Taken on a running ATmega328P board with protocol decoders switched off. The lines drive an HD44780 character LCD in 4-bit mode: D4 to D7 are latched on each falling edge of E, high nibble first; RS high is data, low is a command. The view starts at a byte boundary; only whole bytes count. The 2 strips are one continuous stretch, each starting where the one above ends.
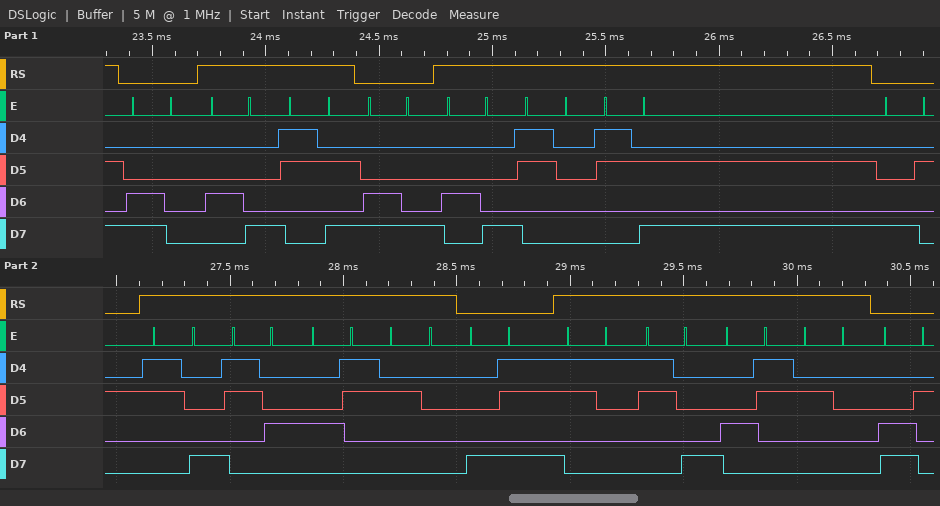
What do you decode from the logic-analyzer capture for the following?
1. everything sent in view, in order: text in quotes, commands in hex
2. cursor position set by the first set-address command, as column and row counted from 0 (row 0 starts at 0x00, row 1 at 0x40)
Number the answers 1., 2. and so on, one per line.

1. 0xC0 "H:" 0xC8 "H0:" 0x82 "84C " 0x8B "18C " 0xC2
2. column 0, row 1
